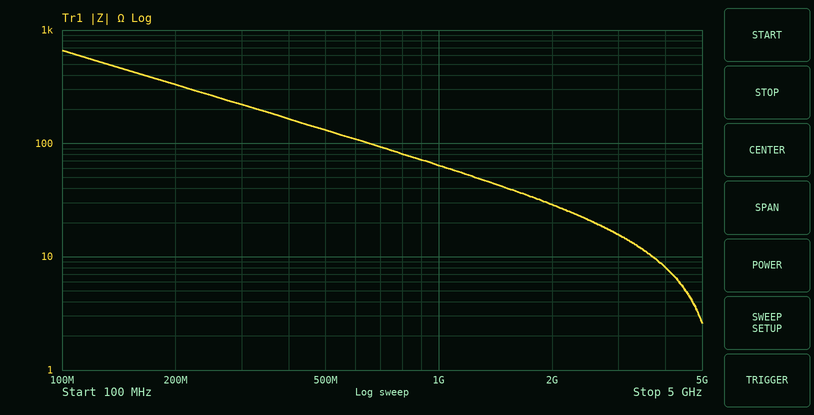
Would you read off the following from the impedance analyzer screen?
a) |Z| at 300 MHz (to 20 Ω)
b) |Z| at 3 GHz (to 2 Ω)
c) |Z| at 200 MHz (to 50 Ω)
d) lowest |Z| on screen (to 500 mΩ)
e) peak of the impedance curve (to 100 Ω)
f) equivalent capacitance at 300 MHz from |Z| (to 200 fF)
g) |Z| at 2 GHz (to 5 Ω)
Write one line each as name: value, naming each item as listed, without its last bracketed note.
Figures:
|Z| at 300 MHz: 220 Ω
|Z| at 3 GHz: 16 Ω
|Z| at 200 MHz: 350 Ω
lowest |Z| on screen: 2.5 Ω
peak of the impedance curve: 700 Ω
equivalent capacitance at 300 MHz from |Z|: 2.4 pF
|Z| at 2 GHz: 30 Ω
